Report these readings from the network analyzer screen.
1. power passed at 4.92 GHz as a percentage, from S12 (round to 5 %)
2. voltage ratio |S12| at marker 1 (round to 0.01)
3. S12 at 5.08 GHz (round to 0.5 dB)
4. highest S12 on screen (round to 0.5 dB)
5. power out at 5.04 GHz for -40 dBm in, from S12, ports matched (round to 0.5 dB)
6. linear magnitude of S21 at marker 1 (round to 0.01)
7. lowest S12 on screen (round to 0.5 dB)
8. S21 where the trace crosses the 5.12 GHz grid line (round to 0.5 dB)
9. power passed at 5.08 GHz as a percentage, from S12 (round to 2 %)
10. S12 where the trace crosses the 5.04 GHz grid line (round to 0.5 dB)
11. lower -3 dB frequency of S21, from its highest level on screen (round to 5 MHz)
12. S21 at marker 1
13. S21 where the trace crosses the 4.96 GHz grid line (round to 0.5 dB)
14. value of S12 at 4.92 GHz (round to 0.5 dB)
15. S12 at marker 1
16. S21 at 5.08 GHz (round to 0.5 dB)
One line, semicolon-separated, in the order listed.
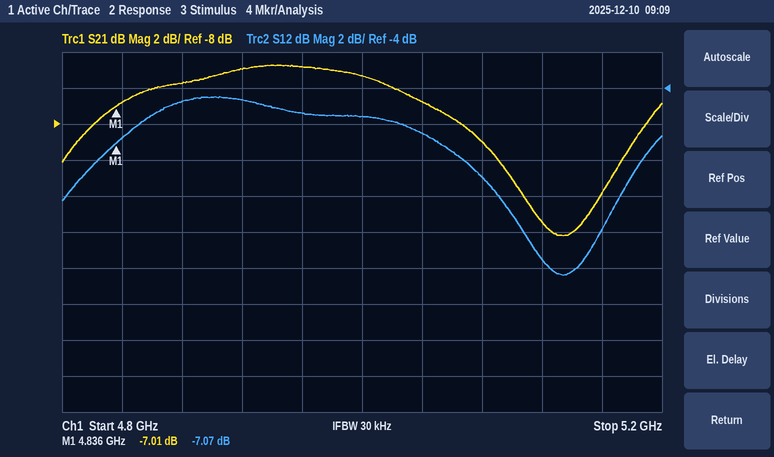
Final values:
35 %; 0.44; -9.0 dB; -4.5 dB; -46.5 dBm; 0.45; -14.5 dB; -13.5 dB; 12 %; -6.5 dB; 4.825 GHz; -7.01 dB; -5.0 dB; -4.5 dB; -7.07 dB; -9.0 dB
